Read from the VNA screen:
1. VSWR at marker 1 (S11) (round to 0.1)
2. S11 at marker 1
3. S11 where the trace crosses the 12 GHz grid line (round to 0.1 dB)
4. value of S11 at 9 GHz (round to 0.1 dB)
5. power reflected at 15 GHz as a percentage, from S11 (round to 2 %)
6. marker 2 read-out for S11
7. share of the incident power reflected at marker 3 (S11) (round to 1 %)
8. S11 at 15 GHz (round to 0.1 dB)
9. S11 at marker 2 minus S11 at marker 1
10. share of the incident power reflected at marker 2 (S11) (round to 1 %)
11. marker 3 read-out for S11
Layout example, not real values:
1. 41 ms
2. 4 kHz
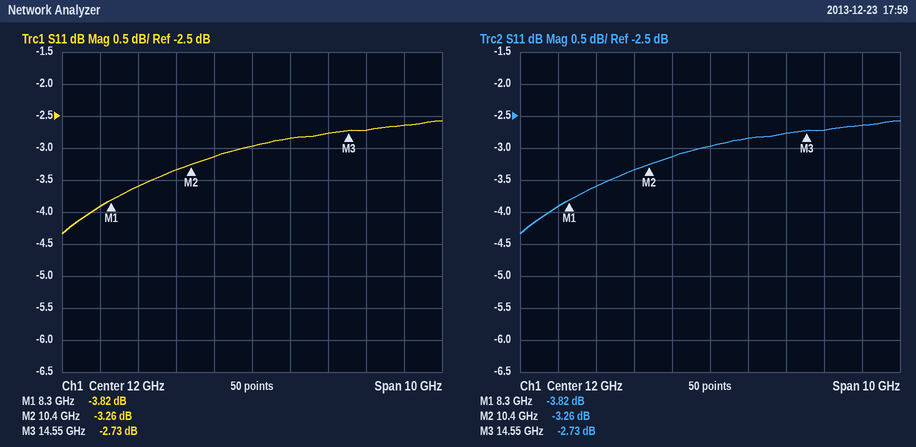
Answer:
1. 4.6
2. -3.82 dB
3. -3.0 dB
4. -3.6 dB
5. 54 %
6. -3.26 dB
7. 53 %
8. -2.7 dB
9. 0.56 dB
10. 47 %
11. -2.73 dB
